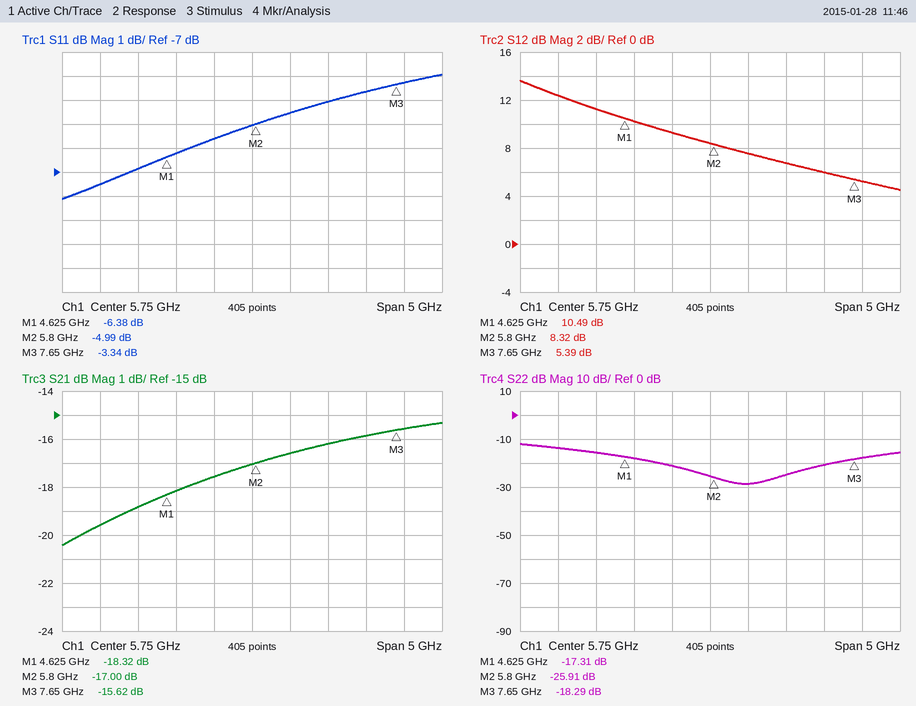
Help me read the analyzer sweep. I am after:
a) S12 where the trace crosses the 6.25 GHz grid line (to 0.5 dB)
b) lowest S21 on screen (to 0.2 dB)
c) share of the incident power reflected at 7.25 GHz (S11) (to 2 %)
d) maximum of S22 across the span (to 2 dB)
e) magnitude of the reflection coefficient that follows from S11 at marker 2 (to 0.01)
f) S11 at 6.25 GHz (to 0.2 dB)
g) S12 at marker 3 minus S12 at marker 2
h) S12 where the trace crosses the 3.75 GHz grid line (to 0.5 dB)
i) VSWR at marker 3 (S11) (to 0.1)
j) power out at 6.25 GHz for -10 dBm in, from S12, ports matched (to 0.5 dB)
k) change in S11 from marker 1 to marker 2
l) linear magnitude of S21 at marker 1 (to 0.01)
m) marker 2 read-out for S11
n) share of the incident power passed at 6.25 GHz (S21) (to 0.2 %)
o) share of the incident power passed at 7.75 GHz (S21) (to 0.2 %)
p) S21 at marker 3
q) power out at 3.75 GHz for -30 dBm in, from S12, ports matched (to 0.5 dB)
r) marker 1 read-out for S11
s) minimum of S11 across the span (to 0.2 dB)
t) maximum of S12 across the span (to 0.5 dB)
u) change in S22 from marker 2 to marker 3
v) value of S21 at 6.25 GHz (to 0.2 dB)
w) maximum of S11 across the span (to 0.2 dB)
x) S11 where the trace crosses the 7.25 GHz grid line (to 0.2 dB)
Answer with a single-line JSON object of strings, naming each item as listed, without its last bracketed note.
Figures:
{"S12 where the trace crosses the 6.25 GHz grid line": "7.5 dB", "lowest S21 on screen": "-20.4 dB", "share of the incident power reflected at 7.25 GHz (S11)": "44 %", "maximum of S22 across the span": "-12 dB", "magnitude of the reflection coefficient that follows from S11 at marker 2": "0.56", "S11 at 6.25 GHz": "-4.6 dB", "S12 at marker 3 minus S12 at marker 2": "-2.93 dB", "S12 where the trace crosses the 3.75 GHz grid line": "12.5 dB", "VSWR at marker 3 (S11)": "5.3", "power out at 6.25 GHz for -10 dBm in, from S12, ports matched": "-2.5 dBm", "change in S11 from marker 1 to marker 2": "1.39 dB", "linear magnitude of S21 at marker 1": "0.12", "marker 2 read-out for S11": "-4.99 dB", "share of the incident power passed at 6.25 GHz (S21)": "2.2 %", "share of the incident power passed at 7.75 GHz (S21)": "2.8 %", "S21 at marker 3": "-15.62 dB", "power out at 3.75 GHz for -30 dBm in, from S12, ports matched": "-17.5 dBm", "marker 1 read-out for S11": "-6.38 dB", "minimum of S11 across the span": "-8.2 dB", "maximum of S12 across the span": "13.5 dB", "change in S22 from marker 2 to marker 3": "7.62 dB", "value of S21 at 6.25 GHz": "-16.6 dB", "maximum of S11 across the span": "-3.0 dB", "S11 where the trace crosses the 7.25 GHz grid line": "-3.6 dB"}
